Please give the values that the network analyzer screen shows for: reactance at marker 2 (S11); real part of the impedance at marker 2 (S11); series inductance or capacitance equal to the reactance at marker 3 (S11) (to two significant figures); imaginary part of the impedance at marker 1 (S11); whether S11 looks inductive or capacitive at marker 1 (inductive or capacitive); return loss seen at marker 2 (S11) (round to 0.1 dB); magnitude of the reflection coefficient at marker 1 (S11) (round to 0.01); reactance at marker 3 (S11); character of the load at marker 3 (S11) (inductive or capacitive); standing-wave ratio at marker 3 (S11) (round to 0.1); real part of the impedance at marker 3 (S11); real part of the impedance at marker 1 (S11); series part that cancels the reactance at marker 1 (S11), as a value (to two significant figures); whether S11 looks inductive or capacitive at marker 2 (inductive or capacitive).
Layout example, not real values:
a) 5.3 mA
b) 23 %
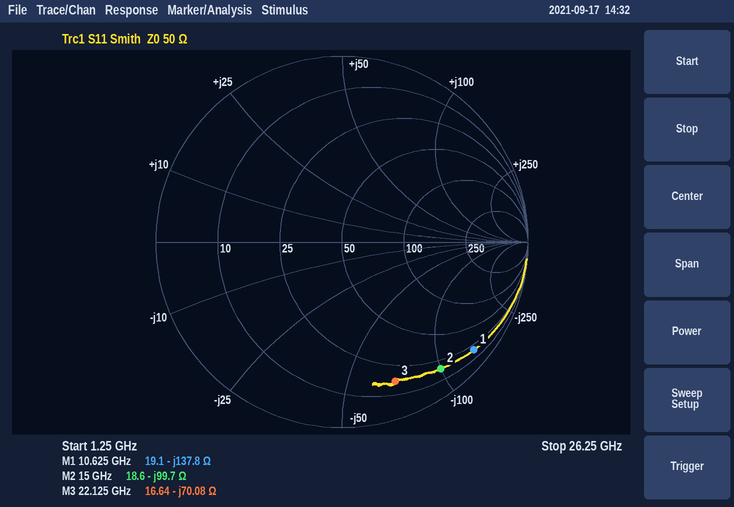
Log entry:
a) -99.7 Ω
b) 18.6 Ω
c) 100 fF
d) -137.8 Ω
e) capacitive
f) 1.3 dB
g) 0.92
h) -70.08 Ω
i) capacitive
j) 9.1
k) 16.64 Ω
l) 19.1 Ω
m) 2.1 nH
n) capacitive
